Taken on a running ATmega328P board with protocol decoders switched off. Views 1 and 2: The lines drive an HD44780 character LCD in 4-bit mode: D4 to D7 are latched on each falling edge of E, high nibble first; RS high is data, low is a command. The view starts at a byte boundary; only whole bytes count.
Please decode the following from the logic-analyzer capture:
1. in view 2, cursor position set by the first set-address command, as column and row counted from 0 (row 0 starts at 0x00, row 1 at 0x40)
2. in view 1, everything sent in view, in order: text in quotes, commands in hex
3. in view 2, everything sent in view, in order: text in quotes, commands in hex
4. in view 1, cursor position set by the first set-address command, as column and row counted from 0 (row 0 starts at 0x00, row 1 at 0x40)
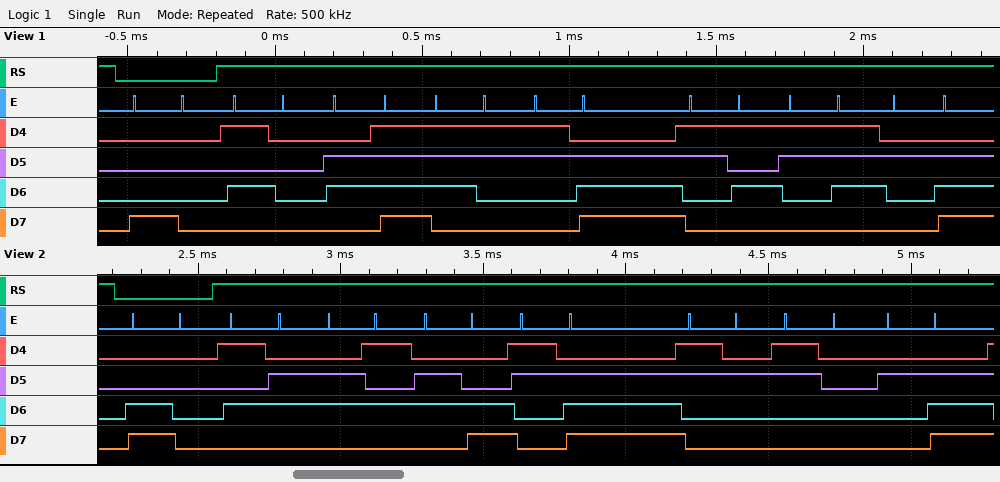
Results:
column 0, row 1
0x80 "Pos>57."
0xC0 "Vel>20."
column 0, row 0
